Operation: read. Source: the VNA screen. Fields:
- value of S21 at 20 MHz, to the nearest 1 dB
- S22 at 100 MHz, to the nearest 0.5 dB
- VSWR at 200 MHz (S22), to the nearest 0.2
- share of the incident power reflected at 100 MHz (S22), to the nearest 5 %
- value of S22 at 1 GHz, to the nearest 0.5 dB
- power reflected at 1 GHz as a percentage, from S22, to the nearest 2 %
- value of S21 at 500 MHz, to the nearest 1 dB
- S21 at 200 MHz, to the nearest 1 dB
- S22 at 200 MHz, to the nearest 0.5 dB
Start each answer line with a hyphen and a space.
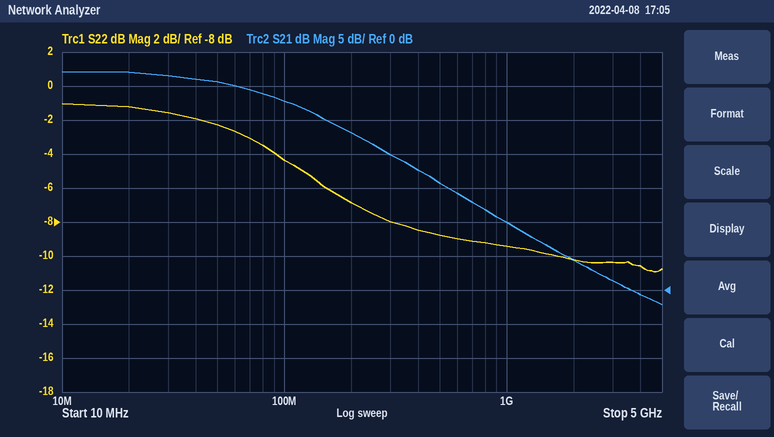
- 32 dB
- -4.5 dB
- 2.6
- 35 %
- -9.5 dB
- 12 %
- 16 dB
- 23 dB
- -7.0 dB
